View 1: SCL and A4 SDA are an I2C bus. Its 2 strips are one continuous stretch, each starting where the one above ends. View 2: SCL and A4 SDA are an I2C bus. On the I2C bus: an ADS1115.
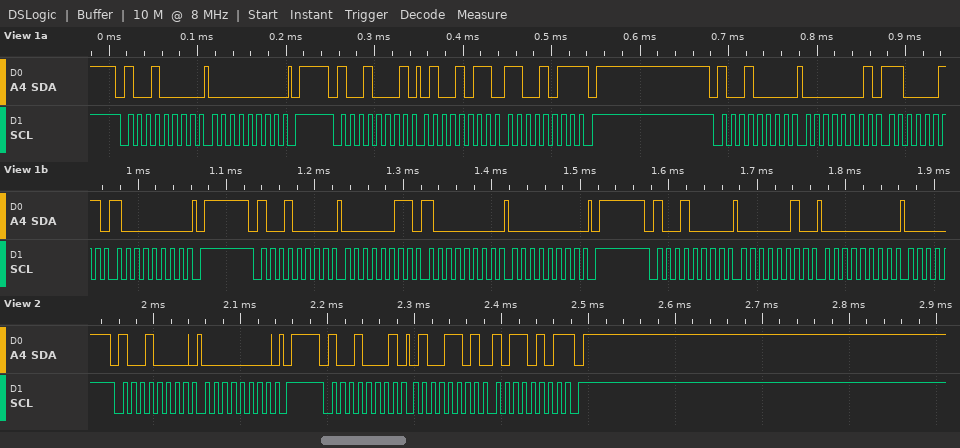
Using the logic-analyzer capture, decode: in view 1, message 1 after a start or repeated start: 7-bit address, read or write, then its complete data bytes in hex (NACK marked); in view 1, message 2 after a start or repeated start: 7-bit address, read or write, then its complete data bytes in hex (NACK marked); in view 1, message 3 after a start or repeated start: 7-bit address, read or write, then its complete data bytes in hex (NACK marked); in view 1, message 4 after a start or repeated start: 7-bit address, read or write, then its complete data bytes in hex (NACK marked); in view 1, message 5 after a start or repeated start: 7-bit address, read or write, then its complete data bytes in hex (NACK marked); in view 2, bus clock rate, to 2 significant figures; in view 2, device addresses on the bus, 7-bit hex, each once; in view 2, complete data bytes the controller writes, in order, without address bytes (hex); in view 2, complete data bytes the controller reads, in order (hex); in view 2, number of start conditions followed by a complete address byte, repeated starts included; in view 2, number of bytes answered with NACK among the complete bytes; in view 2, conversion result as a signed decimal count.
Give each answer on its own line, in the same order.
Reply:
0x48 write: 00
0x48 read: 4B CB NACK
0x48 write: 01 C3 80
0x48 write: 03 80 00
0x48 write: 02 00
100 kHz
0x48
00
4D B5
2
1
19893
